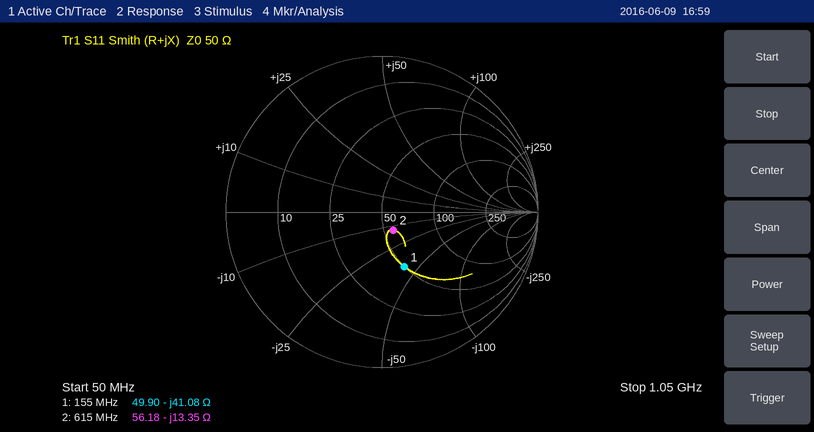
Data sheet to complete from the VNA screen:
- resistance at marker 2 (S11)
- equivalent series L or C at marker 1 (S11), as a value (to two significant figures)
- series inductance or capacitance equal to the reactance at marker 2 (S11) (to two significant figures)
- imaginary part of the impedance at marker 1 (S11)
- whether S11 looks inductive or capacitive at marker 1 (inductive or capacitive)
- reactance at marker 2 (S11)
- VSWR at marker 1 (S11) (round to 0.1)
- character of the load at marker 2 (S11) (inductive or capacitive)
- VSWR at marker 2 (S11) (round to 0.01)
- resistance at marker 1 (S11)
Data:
56.18 Ω
25 pF
19 pF
-41.08 Ω
capacitive
-13.35 Ω
2.2
capacitive
1.32
49.90 Ω
